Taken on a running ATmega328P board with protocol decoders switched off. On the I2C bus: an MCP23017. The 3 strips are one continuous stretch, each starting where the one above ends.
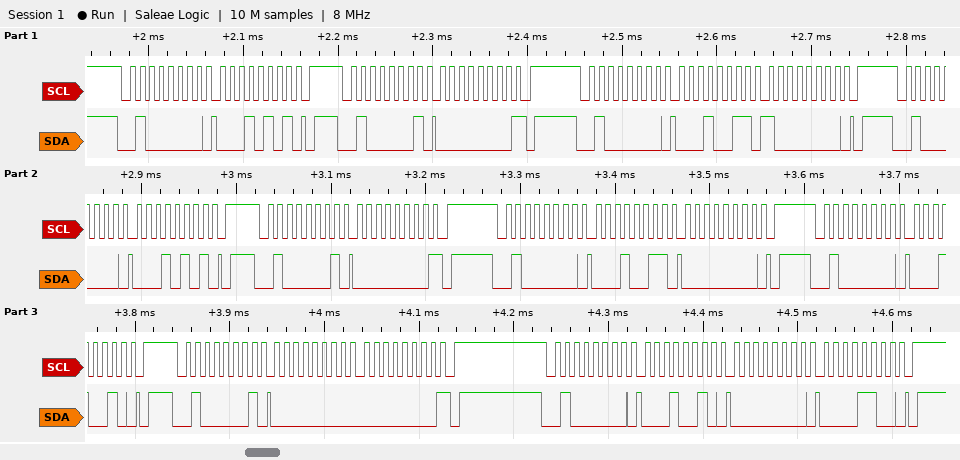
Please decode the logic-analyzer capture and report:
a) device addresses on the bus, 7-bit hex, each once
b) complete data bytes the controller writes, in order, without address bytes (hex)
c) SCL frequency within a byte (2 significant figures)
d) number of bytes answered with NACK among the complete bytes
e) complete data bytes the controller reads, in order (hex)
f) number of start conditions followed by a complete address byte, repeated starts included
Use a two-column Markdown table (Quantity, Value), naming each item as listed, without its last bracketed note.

| Quantity | Value |
|---|---|
| device addresses on the bus, 7-bit hex, each once | 0x20 |
| complete data bytes the controller writes, in order, without address bytes | 15 13 80 15 13 00 12 12 00 0C |
| SCL frequency within a byte | 100 kHz |
| number of bytes answered with NACK among the complete bytes | 3 |
| complete data bytes the controller reads, in order | 00 00 00 00 |
| number of start conditions followed by a complete address byte, repeated starts included | 9 |
